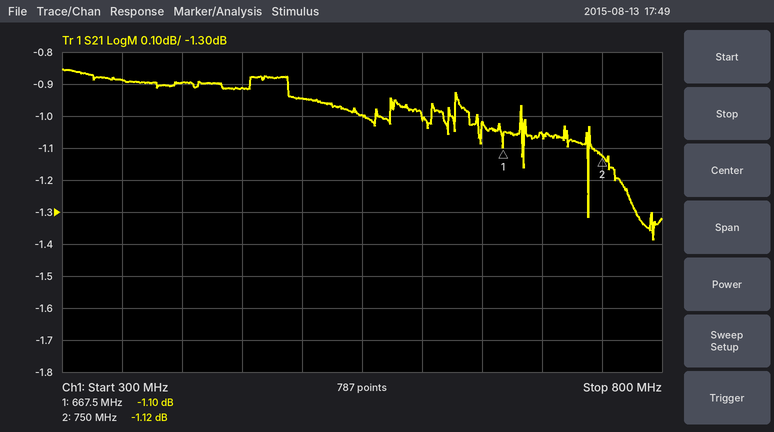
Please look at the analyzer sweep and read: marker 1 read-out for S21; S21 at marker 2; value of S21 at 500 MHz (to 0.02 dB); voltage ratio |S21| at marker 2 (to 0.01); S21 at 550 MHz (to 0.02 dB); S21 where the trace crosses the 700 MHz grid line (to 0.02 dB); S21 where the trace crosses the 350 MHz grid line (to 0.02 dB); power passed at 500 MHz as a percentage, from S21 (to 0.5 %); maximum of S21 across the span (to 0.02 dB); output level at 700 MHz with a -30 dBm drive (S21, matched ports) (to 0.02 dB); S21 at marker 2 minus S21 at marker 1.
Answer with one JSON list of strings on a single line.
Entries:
["-1.10 dB", "-1.12 dB", "-0.94 dB", "0.88", "-1.00 dB", "-1.06 dB", "-0.88 dB", "80.5 %", "-0.86 dB", "-31.06 dBm", "-0.02 dB"]
